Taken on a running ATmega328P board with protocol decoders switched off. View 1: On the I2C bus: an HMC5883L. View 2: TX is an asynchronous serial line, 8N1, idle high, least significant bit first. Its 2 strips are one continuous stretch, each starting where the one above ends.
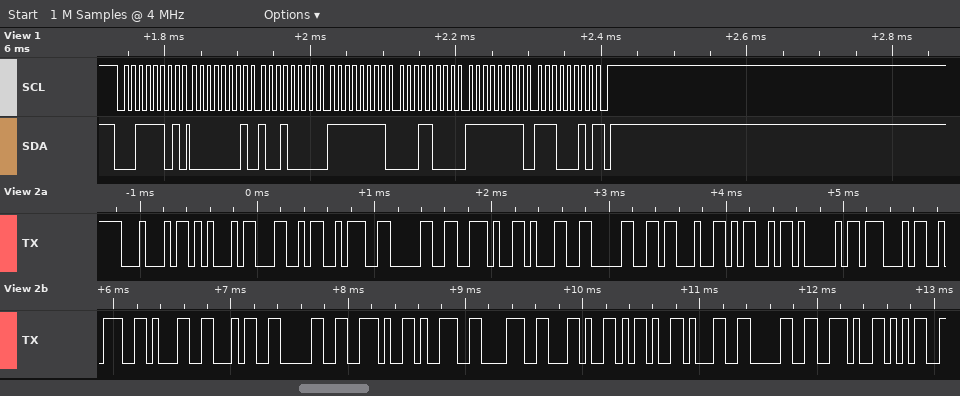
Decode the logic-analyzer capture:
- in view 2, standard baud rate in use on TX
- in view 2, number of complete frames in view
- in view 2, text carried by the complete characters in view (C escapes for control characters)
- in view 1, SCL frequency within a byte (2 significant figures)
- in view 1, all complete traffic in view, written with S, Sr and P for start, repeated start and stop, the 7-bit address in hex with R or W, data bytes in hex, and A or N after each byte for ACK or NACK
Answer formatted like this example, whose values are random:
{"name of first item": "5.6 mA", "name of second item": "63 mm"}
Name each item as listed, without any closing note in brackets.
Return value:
{"in view 2, standard baud rate in use on TX": "19200 baud", "in view 2, number of complete frames in view": "25", "in view 2, text carried by the complete characters in view": "\"DEL:0.10#MAG:140.98,-10.5\"", "in view 1, SCL frequency within a byte": "100 kHz", "in view 1, all complete traffic in view, written with S, Sr and P for start, repeated start and stop, the 7-bit address in hex with R or W, data bytes in hex, and A or N after each byte for ACK or NACK": "S 1ER A 01 A 90 A FF A 18 A FF A E2 N P"}
